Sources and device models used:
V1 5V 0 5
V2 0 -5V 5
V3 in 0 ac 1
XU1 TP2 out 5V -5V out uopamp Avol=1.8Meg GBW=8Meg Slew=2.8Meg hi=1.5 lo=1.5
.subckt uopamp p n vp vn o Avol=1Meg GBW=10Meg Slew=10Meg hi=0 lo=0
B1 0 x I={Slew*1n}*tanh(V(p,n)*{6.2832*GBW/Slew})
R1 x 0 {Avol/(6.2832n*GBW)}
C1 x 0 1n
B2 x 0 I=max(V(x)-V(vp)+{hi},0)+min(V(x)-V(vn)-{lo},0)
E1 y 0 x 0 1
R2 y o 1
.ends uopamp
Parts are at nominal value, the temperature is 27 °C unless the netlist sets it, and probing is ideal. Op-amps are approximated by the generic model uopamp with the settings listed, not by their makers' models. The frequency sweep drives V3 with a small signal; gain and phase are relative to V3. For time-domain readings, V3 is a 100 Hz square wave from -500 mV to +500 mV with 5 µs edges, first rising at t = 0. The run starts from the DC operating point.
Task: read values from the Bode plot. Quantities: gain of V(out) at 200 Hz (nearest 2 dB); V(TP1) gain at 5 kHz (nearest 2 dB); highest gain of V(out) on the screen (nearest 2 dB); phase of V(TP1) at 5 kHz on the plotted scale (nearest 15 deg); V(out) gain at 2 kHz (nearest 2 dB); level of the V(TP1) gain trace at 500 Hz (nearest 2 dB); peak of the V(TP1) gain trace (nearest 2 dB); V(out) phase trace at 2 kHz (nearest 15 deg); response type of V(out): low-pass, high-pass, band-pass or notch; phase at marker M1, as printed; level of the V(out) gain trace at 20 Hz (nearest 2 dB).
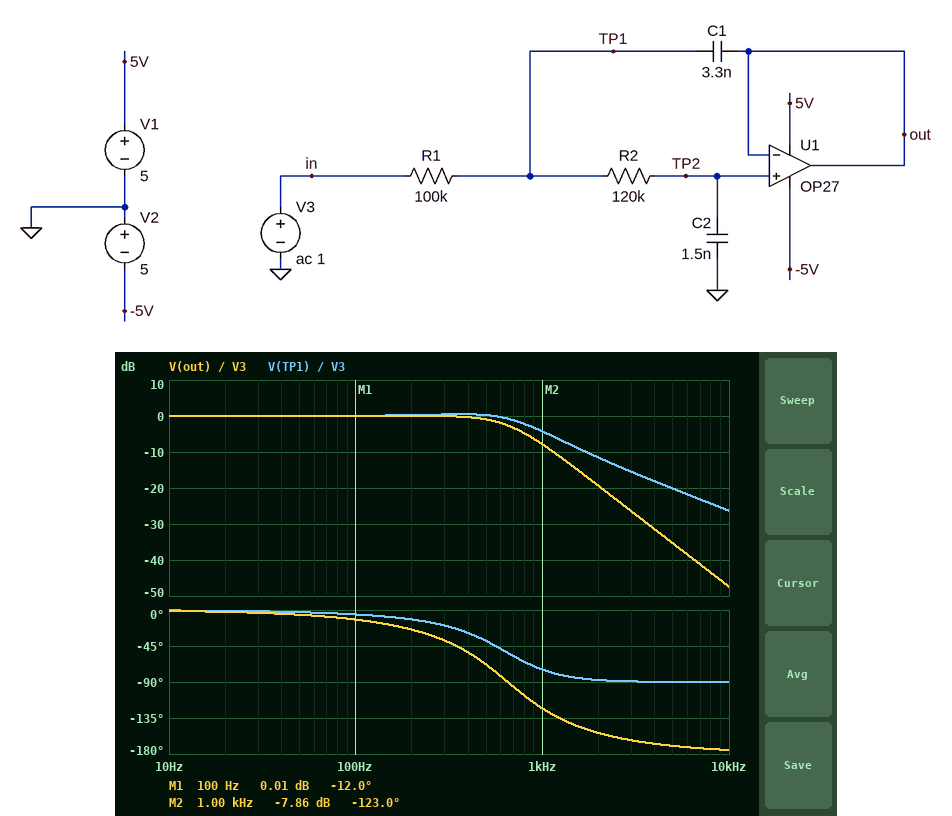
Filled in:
0 dB
-20 dB
0 dB
-90 deg
-20 dB
0 dB
0 dB
-150 deg
low-pass
-12.0 deg
0 dB
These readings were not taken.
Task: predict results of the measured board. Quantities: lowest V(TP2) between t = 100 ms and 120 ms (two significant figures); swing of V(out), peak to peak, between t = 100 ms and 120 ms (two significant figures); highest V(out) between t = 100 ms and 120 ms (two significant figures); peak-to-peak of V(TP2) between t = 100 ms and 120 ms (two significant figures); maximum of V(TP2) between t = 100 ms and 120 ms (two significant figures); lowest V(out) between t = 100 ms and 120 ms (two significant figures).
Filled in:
-560 mV
1.1 V
560 mV
1.1 V
560 mV
-560 mV
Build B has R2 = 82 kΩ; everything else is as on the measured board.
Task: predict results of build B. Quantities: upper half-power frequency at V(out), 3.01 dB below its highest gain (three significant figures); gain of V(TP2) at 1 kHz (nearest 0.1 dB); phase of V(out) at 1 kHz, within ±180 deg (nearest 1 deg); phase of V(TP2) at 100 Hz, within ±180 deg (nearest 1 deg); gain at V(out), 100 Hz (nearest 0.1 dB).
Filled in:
820 Hz
-5.2 dB
-109 deg
-10 deg
0 dB
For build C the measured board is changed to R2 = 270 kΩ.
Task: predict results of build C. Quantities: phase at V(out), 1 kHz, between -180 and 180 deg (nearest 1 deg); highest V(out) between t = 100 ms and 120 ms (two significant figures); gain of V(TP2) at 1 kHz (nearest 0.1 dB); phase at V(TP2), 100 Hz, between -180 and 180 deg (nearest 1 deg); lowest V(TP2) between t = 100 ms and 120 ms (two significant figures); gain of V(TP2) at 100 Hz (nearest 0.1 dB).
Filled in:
-141 deg
530 mV
-14.8 dB
-20 deg
-530 mV
-0.1 dB
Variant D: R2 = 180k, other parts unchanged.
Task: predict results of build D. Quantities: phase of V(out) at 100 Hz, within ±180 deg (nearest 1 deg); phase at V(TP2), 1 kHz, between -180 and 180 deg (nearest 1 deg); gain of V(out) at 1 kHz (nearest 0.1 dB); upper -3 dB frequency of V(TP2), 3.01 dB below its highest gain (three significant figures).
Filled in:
-15 deg
-134 deg
-11.2 dB
536 Hz
